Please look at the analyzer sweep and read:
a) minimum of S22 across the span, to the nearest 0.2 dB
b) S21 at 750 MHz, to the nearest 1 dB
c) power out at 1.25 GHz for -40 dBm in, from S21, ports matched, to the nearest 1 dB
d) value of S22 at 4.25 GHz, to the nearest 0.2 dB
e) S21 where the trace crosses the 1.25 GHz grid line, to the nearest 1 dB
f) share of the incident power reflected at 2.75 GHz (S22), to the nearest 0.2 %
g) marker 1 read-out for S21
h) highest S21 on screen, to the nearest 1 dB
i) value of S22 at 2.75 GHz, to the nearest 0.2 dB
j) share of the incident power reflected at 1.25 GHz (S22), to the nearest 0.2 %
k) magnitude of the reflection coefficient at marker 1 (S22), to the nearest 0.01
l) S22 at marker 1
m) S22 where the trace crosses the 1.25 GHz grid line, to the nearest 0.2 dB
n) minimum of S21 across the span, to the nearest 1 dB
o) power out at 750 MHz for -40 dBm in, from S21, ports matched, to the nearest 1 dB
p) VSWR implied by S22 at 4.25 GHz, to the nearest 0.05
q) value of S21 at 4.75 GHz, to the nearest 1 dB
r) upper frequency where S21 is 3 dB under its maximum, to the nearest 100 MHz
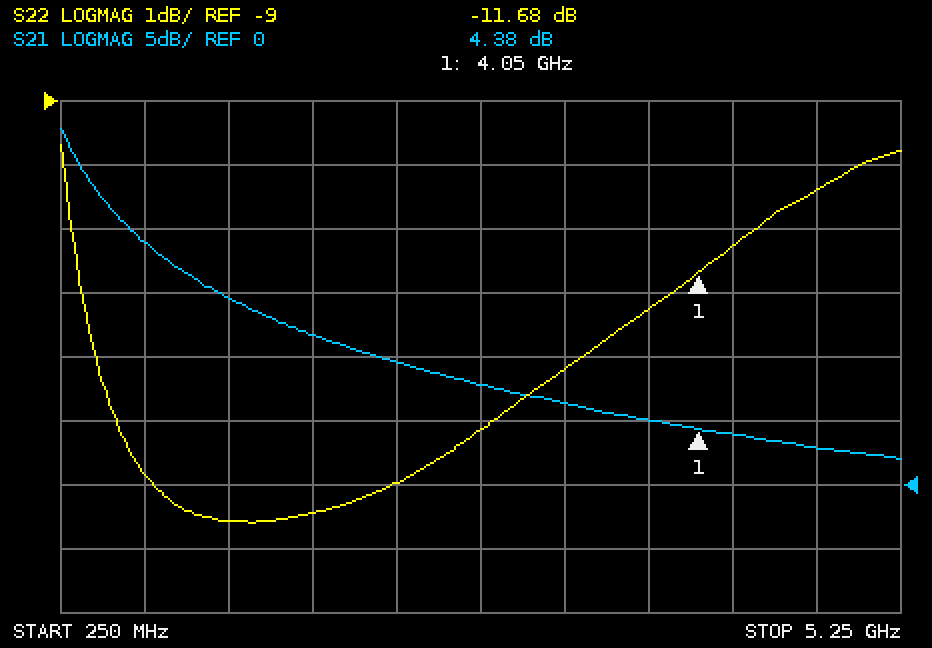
-15.6 dB
19 dB
-25 dBm
-11.2 dB
15 dB
3.8 %
4.38 dB
28 dB
-14.2 dB
2.8 %
0.26
-11.68 dB
-15.6 dB
2 dB
-21 dBm
1.75
3 dB
400 MHz
